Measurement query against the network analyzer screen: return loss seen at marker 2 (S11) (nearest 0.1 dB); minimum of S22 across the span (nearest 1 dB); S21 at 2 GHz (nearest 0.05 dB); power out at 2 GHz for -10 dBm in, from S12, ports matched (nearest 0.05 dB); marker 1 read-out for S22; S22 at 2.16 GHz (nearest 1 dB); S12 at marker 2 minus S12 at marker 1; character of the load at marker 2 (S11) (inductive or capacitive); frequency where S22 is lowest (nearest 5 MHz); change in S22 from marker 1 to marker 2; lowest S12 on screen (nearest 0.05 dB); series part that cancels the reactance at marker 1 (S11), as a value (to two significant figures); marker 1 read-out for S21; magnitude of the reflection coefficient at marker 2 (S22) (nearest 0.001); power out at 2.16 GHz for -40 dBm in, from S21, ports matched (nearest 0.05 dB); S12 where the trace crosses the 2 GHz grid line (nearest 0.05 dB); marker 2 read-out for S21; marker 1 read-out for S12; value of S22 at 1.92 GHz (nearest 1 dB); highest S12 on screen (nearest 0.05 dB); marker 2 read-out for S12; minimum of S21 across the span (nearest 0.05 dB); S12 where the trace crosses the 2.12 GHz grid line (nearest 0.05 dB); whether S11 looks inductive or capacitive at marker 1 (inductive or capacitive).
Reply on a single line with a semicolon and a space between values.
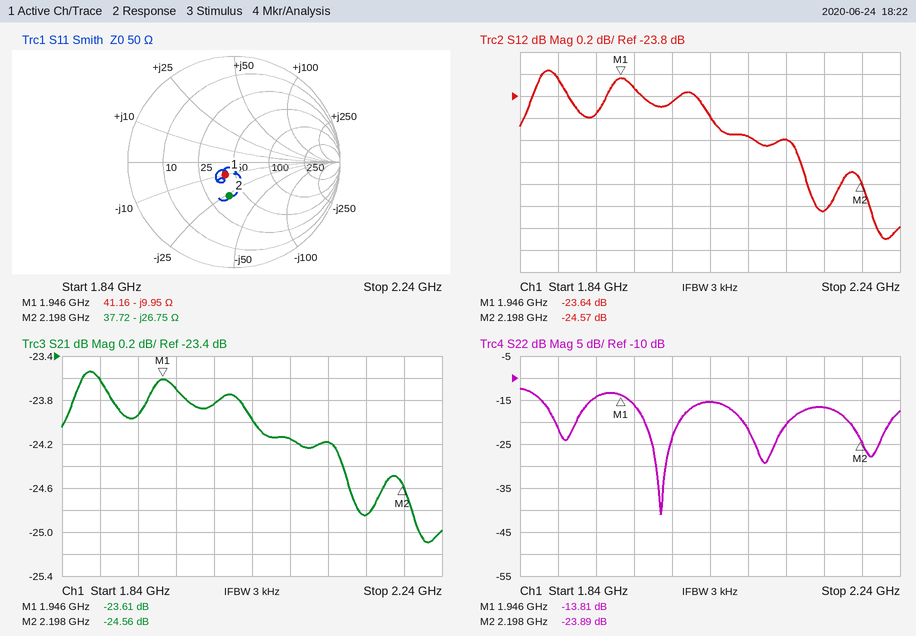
9.9 dB; -41 dB; -23.85 dB; -33.85 dBm; -13.81 dB; -17 dB; -0.93 dB; capacitive; 1.990 GHz; -10.08 dB; -25.10 dB; 810 pH; -23.61 dB; 0.064; -64.85 dBm; -23.85 dB; -24.56 dB; -23.64 dB; -14 dB; -23.55 dB; -24.57 dB; -25.10 dB; -24.20 dB; capacitive
